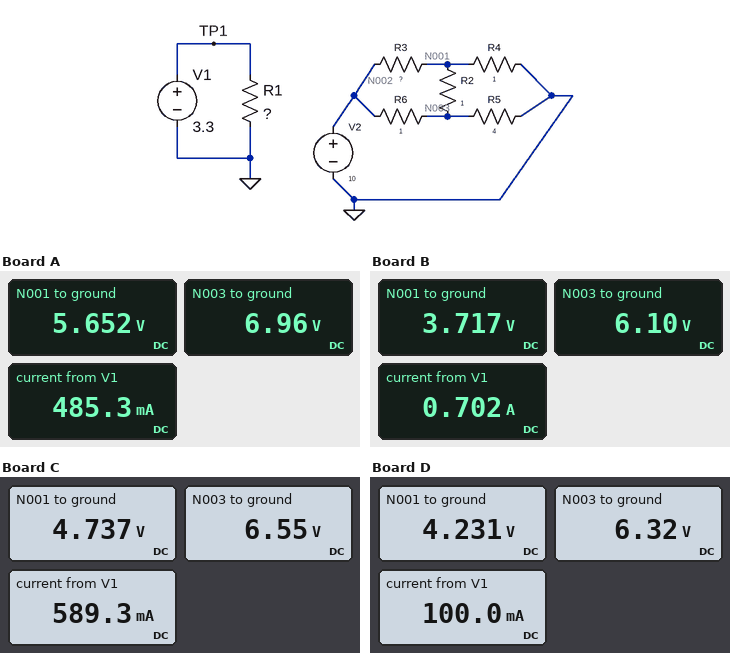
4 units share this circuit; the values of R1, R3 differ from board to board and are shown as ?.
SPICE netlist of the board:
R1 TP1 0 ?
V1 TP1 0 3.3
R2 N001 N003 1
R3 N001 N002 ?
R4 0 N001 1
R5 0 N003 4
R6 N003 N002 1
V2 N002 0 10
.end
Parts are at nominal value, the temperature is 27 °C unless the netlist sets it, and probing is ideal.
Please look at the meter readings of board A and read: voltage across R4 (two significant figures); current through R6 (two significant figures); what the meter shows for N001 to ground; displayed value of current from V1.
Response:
5.7 V
3.0 A
5.652 V
485.3 mA
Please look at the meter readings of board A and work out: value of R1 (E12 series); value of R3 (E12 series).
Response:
6.8 Ω
1 Ω
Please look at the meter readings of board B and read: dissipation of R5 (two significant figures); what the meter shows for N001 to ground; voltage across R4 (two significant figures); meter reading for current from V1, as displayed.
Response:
9.3 W
3.717 V
3.7 V
0.702 A
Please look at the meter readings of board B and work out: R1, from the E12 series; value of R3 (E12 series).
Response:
4.7 Ω
4.7 Ω
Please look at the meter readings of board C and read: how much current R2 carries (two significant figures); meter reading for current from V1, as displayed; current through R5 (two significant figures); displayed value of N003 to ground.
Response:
1.8 A
589.3 mA
1.6 A
6.55 V
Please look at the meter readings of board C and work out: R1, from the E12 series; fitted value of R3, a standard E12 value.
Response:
5.6 Ω
1.8 Ω
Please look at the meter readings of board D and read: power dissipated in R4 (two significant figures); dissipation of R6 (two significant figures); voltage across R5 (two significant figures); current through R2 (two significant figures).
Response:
18 W
14 W
6.3 V
2.1 A
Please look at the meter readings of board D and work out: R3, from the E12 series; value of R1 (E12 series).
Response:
2.7 Ω
33 Ω
